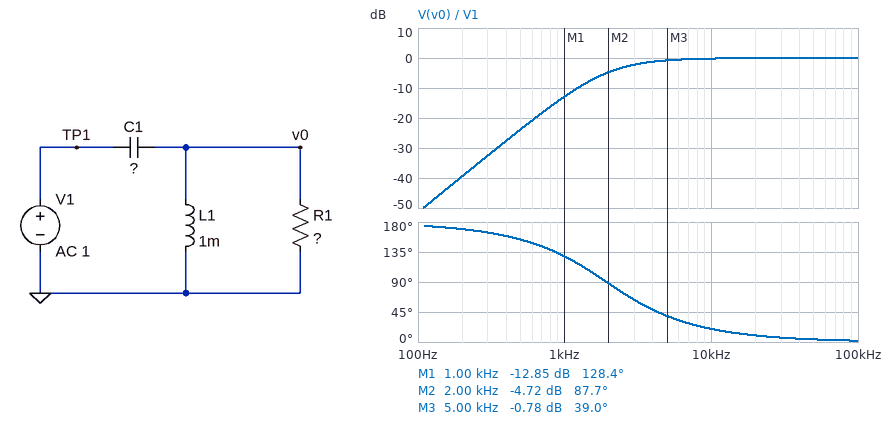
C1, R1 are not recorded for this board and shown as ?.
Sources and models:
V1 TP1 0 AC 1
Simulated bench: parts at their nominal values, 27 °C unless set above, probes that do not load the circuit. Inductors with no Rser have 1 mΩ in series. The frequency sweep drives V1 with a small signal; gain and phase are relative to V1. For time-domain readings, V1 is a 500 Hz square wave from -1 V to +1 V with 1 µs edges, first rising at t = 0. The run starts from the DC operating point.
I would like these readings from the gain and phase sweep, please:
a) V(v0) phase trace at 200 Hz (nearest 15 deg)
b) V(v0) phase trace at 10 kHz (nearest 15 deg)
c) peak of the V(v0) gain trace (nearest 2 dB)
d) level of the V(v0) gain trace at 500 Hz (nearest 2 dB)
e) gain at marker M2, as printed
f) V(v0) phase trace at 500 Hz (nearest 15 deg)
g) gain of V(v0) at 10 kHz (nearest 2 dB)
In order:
165 deg
15 deg
0 dB
-24 dB
-4.72 dB
150 deg
0 dB
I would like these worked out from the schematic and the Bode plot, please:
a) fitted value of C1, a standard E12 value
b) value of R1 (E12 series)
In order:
6.8 µF
6.8 Ω
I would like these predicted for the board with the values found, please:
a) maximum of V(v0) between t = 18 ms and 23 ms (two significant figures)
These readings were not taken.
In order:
2.0 V
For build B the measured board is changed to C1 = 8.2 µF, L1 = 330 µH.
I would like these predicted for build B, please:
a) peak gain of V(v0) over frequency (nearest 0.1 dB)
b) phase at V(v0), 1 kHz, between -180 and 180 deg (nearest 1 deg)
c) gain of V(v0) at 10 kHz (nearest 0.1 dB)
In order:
1.7 dB
161 deg
0.4 dB
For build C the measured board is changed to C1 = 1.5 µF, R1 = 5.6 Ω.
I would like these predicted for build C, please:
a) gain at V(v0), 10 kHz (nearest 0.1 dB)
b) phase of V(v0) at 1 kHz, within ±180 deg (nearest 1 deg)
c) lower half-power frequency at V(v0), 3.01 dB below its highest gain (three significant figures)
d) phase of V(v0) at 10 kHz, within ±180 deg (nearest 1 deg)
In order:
-6.3 dB
130 deg
18.1 kHz
66 deg
